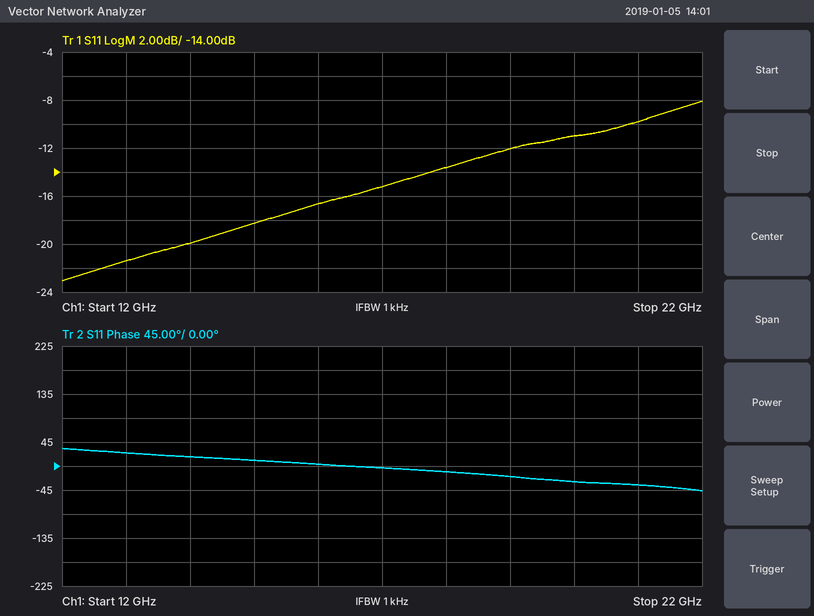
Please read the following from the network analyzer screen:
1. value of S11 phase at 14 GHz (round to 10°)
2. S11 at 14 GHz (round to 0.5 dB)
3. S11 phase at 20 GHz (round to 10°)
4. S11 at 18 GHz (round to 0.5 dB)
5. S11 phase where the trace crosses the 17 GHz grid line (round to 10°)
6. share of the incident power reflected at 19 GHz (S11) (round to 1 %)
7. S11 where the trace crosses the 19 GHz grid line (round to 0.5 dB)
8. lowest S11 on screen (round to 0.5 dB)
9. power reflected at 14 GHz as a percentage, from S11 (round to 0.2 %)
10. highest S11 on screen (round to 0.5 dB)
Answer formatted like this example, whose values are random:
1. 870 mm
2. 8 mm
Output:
1. 20°
2. -20.0 dB
3. -30°
4. -13.5 dB
5. 0°
6. 6 %
7. -12.0 dB
8. -23.0 dB
9. 1.0 %
10. -8.0 dB
